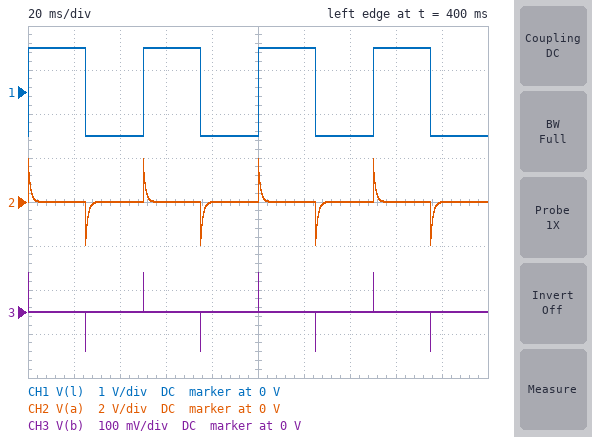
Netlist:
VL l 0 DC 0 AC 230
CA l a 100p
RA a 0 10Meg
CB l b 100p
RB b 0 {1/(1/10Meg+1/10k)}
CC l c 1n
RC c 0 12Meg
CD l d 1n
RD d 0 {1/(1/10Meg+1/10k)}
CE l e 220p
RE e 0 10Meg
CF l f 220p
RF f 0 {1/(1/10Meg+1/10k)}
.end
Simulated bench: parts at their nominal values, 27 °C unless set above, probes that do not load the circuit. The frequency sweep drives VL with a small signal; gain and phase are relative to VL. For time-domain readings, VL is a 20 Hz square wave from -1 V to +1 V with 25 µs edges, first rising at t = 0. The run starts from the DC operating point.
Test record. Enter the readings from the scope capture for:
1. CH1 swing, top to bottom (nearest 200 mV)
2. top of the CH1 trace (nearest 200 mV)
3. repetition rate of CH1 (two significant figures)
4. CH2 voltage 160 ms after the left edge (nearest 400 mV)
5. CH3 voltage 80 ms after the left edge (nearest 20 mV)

2.0 V
1.0 V
20 Hz
0 V
0 V
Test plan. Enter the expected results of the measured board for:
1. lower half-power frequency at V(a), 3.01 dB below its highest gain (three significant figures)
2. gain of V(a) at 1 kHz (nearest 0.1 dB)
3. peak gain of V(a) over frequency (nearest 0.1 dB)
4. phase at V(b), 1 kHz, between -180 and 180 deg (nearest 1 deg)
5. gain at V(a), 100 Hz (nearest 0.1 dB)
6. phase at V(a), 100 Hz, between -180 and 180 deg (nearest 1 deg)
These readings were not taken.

159 Hz
-0.1 dB
0 dB
90 deg
-5.5 dB
58 deg
